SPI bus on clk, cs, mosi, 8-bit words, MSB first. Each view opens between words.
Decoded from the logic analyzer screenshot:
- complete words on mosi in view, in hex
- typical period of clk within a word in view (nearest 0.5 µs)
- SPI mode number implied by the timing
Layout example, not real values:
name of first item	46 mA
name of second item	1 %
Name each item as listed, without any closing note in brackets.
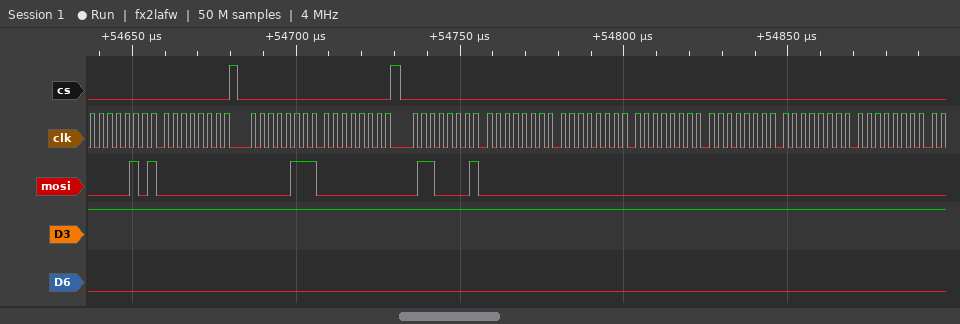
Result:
complete words on mosi in view, in hex	05, 00, 07, 00, 61, 00, 00, 00, 00, 00, 00
typical period of clk within a word in view	2.5 µs
SPI mode number implied by the timing	0
